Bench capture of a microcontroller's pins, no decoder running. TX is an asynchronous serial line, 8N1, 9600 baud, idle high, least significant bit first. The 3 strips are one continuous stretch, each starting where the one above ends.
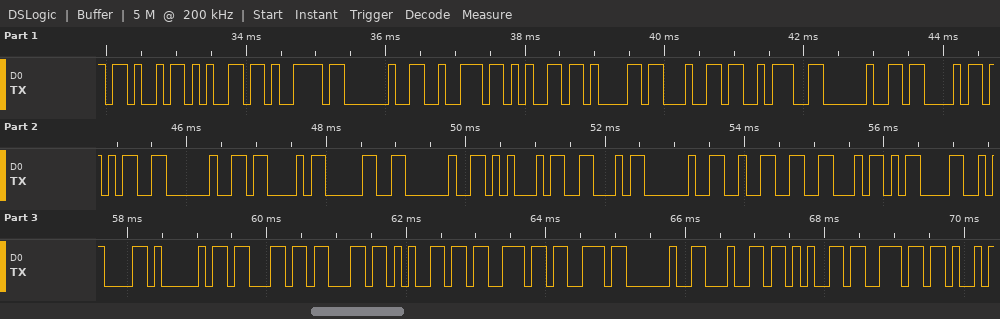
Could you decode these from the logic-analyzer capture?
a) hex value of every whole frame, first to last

0x4B 0x65 0x79 0x20 0x72 0x65 0x61 0x64 0x3A 0x20 0x43 0x35 0x20 0x43 0x30 0x20 0x45 0x46 0x20 0x32 0x46 0x0D 0x0A 0x41 0x63 0x63 0x65 0x73 0x73 0x20 0x64 0x65 0x6E
